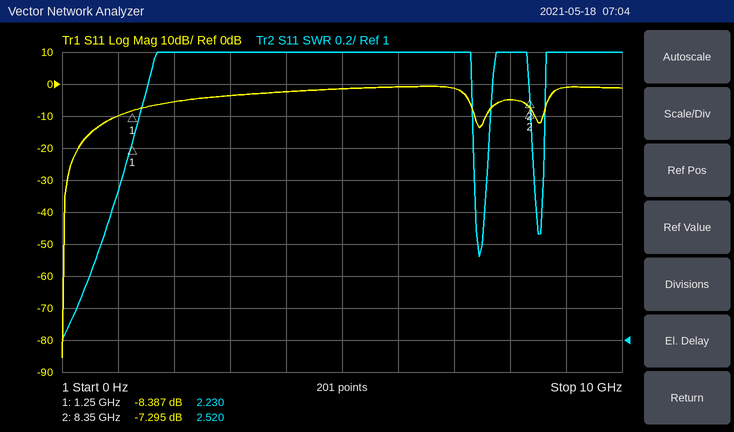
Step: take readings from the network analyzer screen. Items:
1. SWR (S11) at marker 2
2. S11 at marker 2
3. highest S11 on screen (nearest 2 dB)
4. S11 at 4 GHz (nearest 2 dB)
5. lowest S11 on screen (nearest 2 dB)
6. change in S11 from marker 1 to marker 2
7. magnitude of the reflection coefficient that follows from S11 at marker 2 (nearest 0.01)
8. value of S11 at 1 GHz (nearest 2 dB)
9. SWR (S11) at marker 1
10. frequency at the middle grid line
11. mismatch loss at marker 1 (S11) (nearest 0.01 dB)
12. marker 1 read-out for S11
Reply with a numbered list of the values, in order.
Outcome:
1. 2.520
2. -7.295 dB
3. 0 dB
4. -2 dB
5. -86 dB
6. 1.092 dB
7. 0.43
8. -10 dB
9. 2.230
10. 5 GHz
11. 0.68 dB
12. -8.387 dB
